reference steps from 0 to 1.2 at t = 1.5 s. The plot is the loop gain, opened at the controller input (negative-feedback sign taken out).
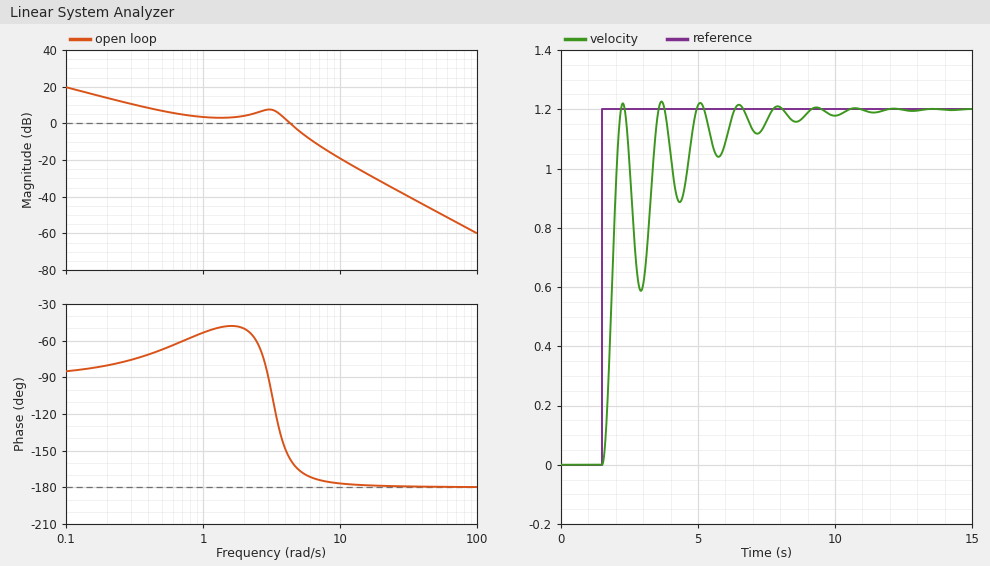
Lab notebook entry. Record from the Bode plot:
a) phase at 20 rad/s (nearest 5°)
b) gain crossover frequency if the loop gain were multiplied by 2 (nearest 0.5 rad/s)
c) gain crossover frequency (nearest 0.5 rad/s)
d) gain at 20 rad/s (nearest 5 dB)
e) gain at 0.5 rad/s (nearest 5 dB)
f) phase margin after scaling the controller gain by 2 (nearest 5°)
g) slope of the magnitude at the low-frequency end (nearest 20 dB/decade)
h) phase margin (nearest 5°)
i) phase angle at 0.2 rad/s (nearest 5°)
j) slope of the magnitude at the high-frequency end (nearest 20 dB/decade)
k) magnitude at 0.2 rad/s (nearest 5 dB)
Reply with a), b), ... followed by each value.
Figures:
a) -180°
b) 5.5 rad/s
c) 4.5 rad/s
d) -30 dB
e) 5 dB
f) 10°
g) -20 dB/decade
h) 25°
i) -80°
j) -40 dB/decade
k) 15 dB
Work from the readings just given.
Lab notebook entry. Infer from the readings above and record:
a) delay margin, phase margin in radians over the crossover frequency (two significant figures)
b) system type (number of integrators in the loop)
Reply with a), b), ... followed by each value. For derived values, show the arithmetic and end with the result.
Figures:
a) 25 × π / 180 / 4.5 = 0.097 s
b) 1
